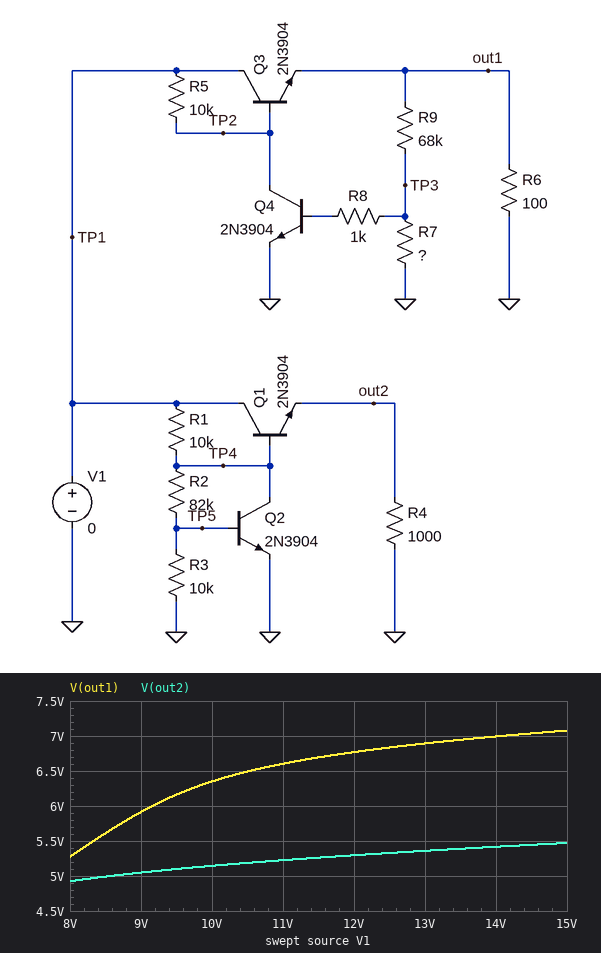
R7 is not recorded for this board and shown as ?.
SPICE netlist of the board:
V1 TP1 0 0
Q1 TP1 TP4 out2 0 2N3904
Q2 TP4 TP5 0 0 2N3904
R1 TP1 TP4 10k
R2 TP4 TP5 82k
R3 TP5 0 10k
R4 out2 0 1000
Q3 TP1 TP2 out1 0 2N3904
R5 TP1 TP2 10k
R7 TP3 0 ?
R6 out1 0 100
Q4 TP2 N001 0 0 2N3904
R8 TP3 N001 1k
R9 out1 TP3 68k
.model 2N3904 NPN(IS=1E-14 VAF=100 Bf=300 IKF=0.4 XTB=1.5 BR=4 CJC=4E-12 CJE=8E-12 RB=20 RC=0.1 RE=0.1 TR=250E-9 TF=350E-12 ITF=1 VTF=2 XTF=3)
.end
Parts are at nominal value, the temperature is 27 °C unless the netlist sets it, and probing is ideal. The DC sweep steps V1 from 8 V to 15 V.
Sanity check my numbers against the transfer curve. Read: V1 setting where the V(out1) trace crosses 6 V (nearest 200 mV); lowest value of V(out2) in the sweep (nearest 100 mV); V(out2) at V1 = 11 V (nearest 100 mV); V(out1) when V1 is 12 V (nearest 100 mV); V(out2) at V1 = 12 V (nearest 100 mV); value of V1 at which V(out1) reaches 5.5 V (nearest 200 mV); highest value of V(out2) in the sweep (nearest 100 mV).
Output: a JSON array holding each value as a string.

["9.2 V", "4.9 V", "5.2 V", "6.8 V", "5.3 V", "8.4 V", "5.5 V"]
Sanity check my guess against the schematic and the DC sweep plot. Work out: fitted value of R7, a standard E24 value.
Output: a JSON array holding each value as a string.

["6.8 kΩ"]
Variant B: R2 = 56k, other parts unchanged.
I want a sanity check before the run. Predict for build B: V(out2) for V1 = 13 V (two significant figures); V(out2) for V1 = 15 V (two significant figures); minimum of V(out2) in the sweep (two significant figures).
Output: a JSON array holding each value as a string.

["3.7 V", "3.8 V", "3.5 V"]
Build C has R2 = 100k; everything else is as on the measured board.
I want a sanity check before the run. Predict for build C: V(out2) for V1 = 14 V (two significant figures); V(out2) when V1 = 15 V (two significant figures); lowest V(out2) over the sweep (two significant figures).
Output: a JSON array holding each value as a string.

["6.5 V", "6.6 V", "5.8 V"]
